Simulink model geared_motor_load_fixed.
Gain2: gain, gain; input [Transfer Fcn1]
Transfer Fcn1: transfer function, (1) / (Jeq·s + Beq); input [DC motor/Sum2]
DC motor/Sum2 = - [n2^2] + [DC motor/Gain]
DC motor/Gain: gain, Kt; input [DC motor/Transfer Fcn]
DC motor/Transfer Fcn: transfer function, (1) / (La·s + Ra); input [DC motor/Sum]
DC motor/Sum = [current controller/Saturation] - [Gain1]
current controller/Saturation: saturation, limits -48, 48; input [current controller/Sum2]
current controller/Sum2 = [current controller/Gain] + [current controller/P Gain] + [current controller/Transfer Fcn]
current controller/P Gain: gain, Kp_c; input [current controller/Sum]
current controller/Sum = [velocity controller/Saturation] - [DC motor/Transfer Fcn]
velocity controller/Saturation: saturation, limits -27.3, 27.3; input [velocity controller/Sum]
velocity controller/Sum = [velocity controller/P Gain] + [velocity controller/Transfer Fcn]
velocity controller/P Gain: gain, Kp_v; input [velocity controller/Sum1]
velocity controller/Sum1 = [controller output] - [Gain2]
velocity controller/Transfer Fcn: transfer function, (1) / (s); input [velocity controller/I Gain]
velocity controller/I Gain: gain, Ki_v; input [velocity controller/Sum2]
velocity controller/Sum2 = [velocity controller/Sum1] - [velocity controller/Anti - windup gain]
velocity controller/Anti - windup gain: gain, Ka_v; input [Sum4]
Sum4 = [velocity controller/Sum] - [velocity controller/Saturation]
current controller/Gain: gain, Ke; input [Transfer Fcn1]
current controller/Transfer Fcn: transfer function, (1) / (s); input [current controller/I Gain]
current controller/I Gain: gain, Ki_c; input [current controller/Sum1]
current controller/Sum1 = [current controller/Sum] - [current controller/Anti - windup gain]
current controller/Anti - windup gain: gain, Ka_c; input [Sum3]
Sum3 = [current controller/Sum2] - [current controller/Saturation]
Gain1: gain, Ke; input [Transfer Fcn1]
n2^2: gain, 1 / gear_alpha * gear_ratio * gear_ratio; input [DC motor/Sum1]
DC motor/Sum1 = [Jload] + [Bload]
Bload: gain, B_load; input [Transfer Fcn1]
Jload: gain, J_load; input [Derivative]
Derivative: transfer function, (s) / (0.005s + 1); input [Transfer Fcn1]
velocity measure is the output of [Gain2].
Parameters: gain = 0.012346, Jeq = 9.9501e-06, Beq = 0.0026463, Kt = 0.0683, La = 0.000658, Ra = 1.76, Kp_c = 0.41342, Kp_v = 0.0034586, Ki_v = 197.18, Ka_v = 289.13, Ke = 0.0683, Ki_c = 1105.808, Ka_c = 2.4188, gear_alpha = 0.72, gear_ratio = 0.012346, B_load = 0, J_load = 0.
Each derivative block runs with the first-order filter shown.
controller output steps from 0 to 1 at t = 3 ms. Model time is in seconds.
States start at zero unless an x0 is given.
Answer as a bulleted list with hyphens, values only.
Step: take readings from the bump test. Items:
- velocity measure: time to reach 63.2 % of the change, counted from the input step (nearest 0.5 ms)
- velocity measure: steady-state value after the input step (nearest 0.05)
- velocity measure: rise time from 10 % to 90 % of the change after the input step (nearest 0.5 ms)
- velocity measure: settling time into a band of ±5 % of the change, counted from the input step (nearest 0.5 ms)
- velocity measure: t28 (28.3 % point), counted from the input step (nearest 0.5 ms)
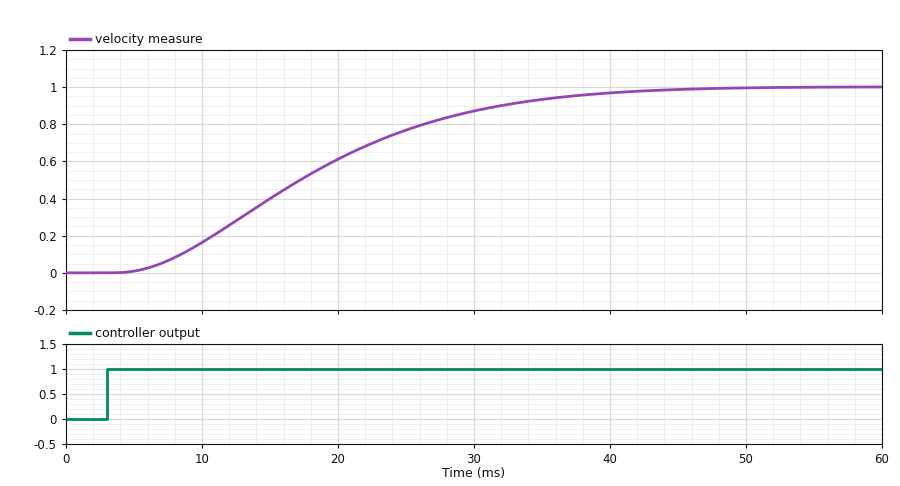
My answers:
- 17.5 ms
- 1.00
- 23.5 ms
- 34.0 ms
- 9.5 ms
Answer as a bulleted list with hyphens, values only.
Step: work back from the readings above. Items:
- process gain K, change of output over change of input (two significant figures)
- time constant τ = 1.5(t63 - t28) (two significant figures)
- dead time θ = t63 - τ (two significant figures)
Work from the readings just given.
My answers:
- 1.0
- 12 ms
- 5.5 ms
